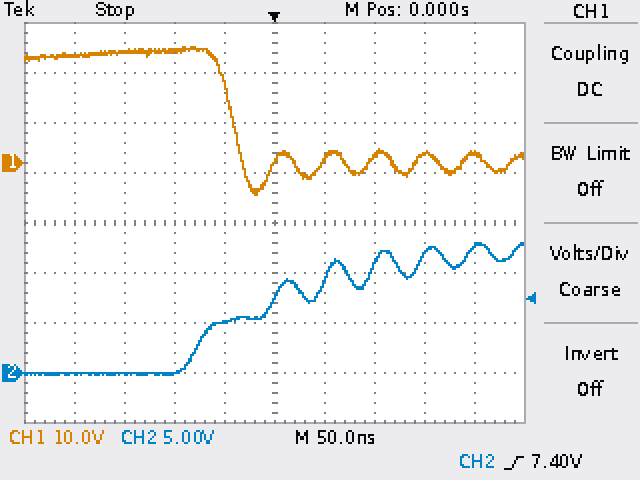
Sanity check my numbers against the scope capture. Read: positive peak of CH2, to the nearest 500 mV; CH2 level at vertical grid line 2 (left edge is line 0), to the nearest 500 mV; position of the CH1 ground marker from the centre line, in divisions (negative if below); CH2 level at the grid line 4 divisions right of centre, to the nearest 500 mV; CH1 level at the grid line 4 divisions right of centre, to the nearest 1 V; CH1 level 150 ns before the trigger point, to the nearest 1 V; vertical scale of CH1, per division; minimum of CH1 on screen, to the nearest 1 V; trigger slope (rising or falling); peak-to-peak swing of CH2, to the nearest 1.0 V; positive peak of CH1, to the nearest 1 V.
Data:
13.0 V
0.0 V
+1.2 div
12.5 V
2 V
22 V
10 V
-6 V
rising
13.0 V
23 V
